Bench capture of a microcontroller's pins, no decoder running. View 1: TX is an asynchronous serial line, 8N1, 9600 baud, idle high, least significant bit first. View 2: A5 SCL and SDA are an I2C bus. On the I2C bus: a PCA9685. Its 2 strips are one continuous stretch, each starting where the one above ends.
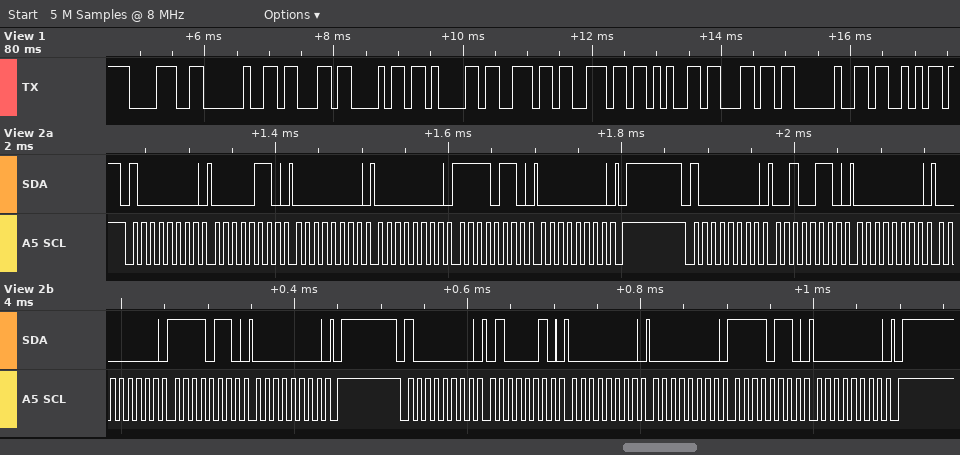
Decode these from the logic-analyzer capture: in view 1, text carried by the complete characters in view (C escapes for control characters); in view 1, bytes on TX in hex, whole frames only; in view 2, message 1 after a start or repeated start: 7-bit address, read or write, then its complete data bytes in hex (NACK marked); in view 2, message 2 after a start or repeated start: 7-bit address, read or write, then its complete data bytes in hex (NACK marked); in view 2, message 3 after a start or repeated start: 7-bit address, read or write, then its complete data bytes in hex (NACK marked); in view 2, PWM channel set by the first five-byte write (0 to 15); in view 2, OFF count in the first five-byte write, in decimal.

"8 channel S"
38 20 63 68 61 6E 6E 65 6C 20 53
0x40 write: 06 00 00 F6 00
0x40 write: 26 00 00 F6 00
0x40 write: 42 00 00 F6 00
0
246
